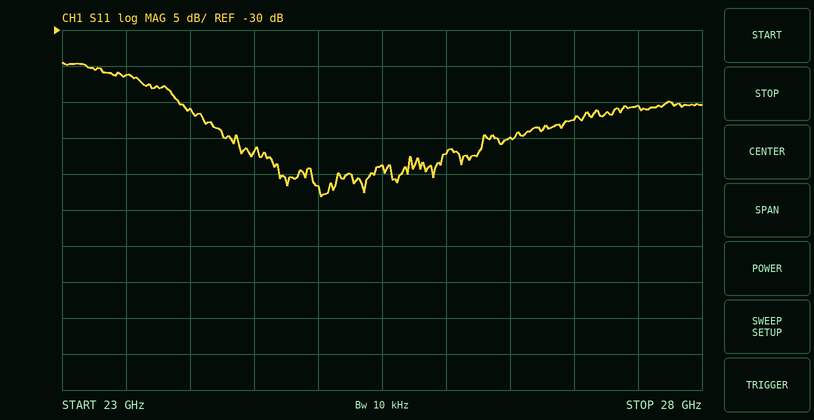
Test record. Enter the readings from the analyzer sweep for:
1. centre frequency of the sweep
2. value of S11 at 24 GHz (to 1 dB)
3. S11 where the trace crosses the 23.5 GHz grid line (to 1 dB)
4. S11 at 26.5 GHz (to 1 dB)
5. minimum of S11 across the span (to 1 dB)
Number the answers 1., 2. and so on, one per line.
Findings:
1. 25.5 GHz
2. -41 dB
3. -36 dB
4. -45 dB
5. -53 dB
